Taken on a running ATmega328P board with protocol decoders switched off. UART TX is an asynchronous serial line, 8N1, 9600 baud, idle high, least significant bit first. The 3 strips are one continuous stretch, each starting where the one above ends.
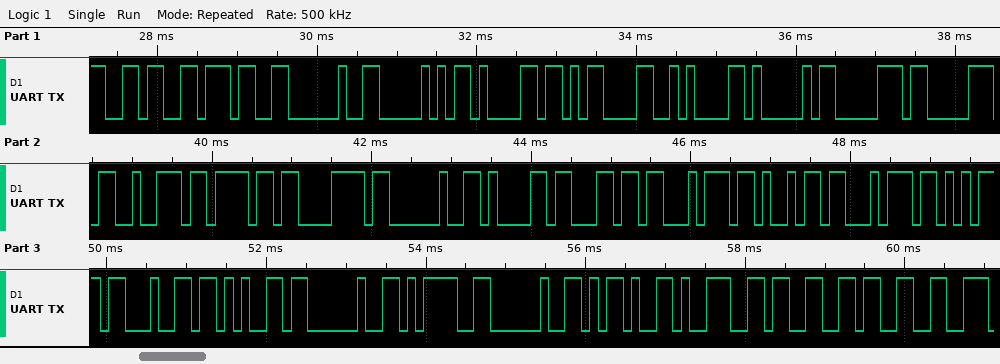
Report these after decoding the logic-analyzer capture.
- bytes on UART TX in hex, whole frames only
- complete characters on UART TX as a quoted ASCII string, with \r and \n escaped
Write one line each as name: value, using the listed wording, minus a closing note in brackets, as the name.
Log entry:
bytes on UART TX in hex, whole frames only: 0x36 0x37 0x20 0x50 0x61 0x0D 0x0A 0x41 0x70 0x70 0x72 0x6F 0x78 0x20 0x61 0x6C 0x74 0x69 0x74 0x75 0x64 0x65 0x20 0x3D 0x20 0x2D 0x39 0x33 0x33
complete characters on UART TX as a quoted ASCII string, with \r and \n escaped: "67 Pa\r\nApprox altitude = -933"
